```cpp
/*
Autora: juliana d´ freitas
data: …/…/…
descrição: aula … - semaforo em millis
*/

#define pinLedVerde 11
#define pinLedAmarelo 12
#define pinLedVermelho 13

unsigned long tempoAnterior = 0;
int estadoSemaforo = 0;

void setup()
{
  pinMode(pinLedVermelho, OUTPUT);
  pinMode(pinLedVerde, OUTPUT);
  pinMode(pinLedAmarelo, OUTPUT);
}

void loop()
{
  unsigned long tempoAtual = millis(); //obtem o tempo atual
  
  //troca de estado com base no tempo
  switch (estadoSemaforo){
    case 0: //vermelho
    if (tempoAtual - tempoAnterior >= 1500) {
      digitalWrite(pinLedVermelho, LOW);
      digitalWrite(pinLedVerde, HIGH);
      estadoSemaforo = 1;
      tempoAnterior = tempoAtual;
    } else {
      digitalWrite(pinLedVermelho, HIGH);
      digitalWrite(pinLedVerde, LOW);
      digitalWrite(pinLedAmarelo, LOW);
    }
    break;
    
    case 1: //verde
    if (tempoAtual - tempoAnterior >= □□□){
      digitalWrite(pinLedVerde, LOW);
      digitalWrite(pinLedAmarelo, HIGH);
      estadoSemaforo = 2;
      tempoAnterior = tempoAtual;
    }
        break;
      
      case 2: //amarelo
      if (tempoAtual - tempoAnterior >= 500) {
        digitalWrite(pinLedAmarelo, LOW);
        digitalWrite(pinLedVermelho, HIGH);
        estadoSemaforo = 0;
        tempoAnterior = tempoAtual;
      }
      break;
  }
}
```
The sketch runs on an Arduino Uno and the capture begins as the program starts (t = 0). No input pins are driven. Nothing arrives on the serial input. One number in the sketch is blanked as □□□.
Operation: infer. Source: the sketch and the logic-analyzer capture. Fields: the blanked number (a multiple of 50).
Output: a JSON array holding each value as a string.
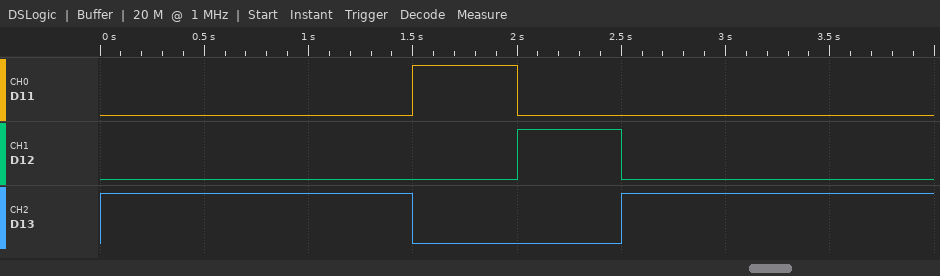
["500"]
